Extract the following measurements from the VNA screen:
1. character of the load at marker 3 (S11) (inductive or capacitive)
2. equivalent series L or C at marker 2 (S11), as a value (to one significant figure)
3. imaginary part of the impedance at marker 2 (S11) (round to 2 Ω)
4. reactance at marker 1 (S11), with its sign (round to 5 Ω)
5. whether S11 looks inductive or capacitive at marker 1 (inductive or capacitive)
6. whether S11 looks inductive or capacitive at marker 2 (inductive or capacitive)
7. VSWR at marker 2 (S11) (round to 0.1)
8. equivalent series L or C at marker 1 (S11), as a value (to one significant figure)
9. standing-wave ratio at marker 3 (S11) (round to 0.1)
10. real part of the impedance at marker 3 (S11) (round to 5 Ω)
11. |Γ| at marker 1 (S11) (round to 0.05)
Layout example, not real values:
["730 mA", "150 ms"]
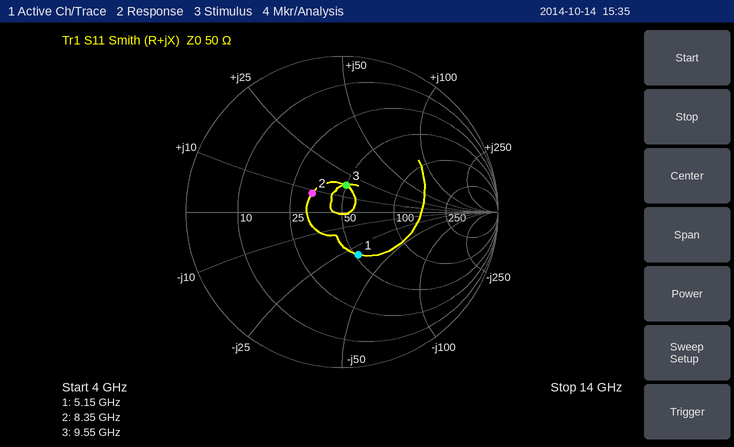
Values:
["inductive", "200 pH", "+8 Ω", "-30 Ω", "capacitive", "inductive", "1.6", "1.0 pF", "1.4", "50 Ω", "0.30"]
